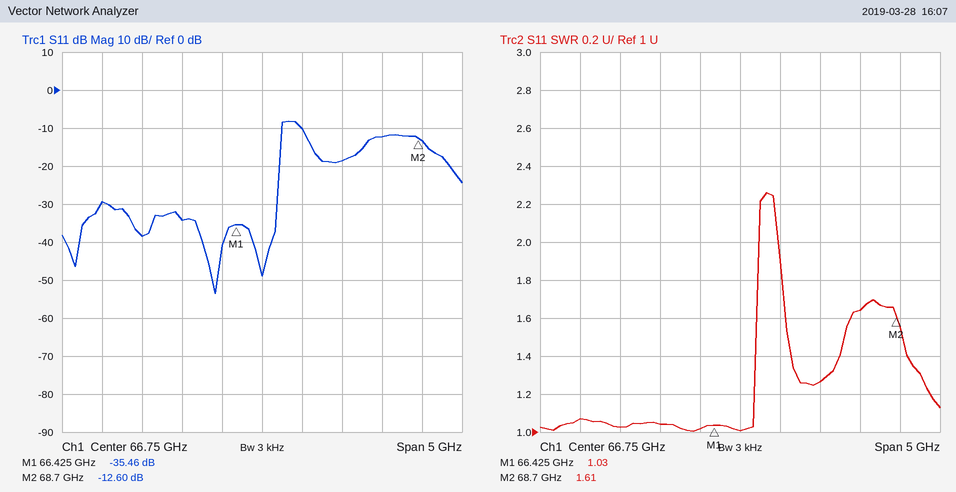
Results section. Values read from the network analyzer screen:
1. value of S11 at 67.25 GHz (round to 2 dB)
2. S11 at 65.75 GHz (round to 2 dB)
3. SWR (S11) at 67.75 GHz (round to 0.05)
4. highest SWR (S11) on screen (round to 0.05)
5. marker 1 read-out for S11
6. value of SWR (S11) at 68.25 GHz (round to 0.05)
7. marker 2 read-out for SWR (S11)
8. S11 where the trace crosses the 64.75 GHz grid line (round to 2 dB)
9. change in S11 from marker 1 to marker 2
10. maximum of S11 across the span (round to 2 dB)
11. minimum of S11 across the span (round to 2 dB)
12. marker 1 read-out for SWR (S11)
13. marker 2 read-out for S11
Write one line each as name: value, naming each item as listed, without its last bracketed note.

value of S11 at 67.25 GHz: -10 dB
S11 at 65.75 GHz: -34 dB
SWR (S11) at 67.75 GHz: 1.25
highest SWR (S11) on screen: 2.25
marker 1 read-out for S11: -35.46 dB
value of SWR (S11) at 68.25 GHz: 1.65
marker 2 read-out for SWR: 1.61
S11 where the trace crosses the 64.75 GHz grid line: -30 dB
change in S11 from marker 1 to marker 2: 22.86 dB
maximum of S11 across the span: -8 dB
minimum of S11 across the span: -54 dB
marker 1 read-out for SWR: 1.03
marker 2 read-out for S11: -12.60 dB
